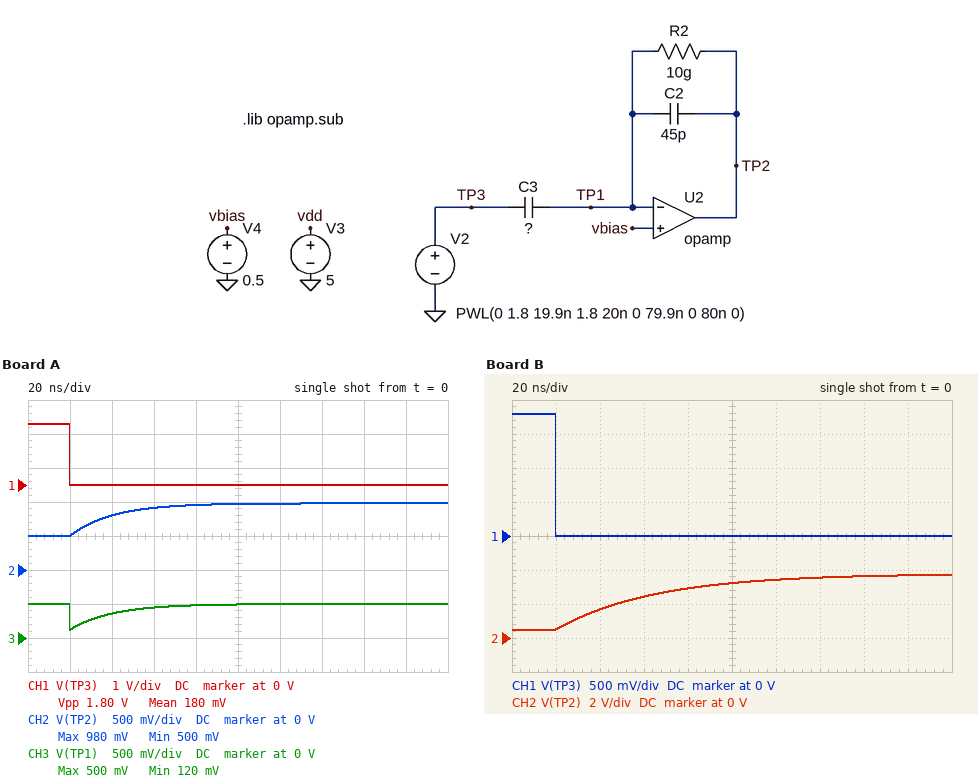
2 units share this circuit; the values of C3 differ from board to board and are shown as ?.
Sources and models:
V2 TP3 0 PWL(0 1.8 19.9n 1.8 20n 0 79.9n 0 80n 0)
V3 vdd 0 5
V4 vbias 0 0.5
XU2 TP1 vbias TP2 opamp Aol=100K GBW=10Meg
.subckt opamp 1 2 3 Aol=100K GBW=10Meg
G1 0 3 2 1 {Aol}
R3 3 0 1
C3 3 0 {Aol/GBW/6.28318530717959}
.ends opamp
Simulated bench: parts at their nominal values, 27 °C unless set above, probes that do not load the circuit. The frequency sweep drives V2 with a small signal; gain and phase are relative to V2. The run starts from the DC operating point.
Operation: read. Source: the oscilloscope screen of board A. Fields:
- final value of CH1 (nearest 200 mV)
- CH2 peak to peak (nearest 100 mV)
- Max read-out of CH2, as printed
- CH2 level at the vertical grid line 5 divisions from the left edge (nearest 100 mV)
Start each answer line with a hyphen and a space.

- 0 V
- 500 mV
- 980 mV
- 1.0 V
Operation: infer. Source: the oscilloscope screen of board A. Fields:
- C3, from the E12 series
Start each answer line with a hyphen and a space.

- 12 pF
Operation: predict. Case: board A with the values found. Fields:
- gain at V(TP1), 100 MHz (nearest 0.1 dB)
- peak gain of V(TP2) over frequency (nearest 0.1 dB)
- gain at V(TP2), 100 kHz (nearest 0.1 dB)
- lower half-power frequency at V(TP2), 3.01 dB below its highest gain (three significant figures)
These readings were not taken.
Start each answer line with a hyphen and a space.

- -13.6 dB
- -11.5 dB
- -11.5 dB
- 354 mHz
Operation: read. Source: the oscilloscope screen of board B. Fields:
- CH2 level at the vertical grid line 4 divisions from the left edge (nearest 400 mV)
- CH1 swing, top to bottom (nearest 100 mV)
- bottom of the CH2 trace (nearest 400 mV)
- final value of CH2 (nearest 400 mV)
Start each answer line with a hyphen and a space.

- 2.8 V
- 1.8 V
- 400 mV
- 3.6 V
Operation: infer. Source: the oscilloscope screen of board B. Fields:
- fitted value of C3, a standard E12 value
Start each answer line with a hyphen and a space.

- 82 pF
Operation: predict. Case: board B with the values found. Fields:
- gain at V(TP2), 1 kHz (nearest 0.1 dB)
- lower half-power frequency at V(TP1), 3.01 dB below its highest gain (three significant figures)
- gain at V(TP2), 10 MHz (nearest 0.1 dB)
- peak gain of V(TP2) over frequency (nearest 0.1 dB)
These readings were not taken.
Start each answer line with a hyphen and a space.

- 5.2 dB
- 3.54 MHz
- -4.3 dB
- 5.2 dB
